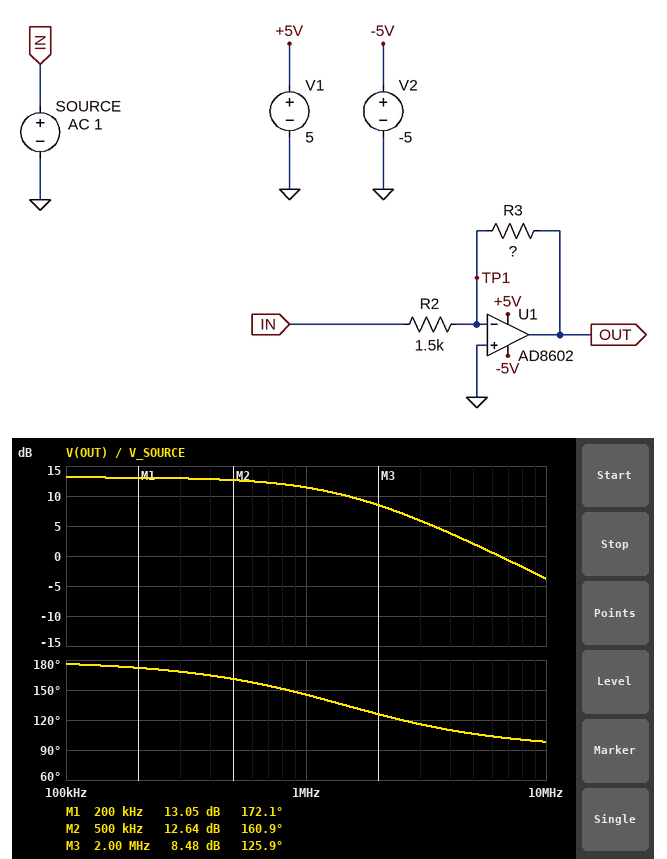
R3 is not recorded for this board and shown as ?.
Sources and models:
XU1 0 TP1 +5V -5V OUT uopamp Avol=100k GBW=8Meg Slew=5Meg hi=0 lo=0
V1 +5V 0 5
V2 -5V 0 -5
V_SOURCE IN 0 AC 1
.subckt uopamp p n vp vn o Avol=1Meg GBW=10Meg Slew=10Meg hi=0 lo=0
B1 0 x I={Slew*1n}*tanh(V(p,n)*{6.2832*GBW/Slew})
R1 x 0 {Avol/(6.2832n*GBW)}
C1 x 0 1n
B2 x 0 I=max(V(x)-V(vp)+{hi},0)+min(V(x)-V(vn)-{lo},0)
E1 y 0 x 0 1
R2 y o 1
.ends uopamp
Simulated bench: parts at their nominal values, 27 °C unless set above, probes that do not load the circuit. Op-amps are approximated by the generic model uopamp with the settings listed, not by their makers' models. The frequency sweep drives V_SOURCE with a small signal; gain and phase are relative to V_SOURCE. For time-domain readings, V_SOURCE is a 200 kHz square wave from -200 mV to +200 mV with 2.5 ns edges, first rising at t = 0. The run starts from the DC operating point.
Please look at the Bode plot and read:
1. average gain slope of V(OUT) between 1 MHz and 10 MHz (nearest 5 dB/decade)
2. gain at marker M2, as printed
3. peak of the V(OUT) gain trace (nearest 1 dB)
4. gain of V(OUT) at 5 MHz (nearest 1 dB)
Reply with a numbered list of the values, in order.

1. -15 dB/decade
2. 12.64 dB
3. 13 dB
4. 2 dB
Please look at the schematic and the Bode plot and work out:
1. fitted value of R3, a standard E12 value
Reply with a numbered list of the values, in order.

1. 6.8 kΩ
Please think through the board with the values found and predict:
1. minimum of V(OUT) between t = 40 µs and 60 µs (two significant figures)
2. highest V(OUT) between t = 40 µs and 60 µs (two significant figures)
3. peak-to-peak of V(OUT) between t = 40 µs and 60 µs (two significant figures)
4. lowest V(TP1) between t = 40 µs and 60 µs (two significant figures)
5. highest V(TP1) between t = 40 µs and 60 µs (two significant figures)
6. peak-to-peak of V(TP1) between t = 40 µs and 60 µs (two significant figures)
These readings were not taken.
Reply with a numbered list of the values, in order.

1. -910 mV
2. 910 mV
3. 1.8 V
4. -330 mV
5. 330 mV
6. 650 mV
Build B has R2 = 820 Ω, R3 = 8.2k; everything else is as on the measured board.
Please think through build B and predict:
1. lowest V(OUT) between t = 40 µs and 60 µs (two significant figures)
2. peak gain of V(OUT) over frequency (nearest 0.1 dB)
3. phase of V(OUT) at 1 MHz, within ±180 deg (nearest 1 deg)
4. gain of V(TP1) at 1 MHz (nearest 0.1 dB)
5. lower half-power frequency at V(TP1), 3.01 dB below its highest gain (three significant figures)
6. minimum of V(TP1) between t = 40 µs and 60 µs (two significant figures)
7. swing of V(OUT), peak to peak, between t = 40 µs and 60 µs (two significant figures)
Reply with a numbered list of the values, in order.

1. -2.0 V
2. 20.0 dB
3. 126 deg
4. -2.7 dB
5. 727 kHz
6. -360 mV
7. 4.0 V
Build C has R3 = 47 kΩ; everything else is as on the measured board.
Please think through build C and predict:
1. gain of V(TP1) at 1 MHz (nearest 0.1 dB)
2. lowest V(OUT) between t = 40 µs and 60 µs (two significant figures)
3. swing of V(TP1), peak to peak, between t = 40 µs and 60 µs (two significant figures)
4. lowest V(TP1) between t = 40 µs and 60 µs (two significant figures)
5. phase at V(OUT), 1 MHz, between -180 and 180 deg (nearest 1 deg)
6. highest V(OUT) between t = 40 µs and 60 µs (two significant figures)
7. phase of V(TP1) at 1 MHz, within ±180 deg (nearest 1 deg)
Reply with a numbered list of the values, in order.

1. -0.5 dB
2. -5.0 V
3. 700 mV
4. -350 mV
5. 104 deg
6. 5.0 V
7. 14 deg
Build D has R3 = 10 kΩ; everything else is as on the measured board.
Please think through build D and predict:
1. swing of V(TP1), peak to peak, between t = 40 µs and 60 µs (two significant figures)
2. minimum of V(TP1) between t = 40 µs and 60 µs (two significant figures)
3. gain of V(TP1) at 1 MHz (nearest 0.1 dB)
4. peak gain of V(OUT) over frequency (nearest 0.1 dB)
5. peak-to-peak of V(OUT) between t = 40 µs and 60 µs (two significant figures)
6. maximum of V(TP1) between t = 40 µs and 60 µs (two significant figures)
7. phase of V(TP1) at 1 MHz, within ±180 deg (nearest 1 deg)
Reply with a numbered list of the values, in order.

1. 690 mV
2. -350 mV
3. -4.4 dB
4. 16.5 dB
5. 2.7 V
6. 350 mV
7. 46 deg
